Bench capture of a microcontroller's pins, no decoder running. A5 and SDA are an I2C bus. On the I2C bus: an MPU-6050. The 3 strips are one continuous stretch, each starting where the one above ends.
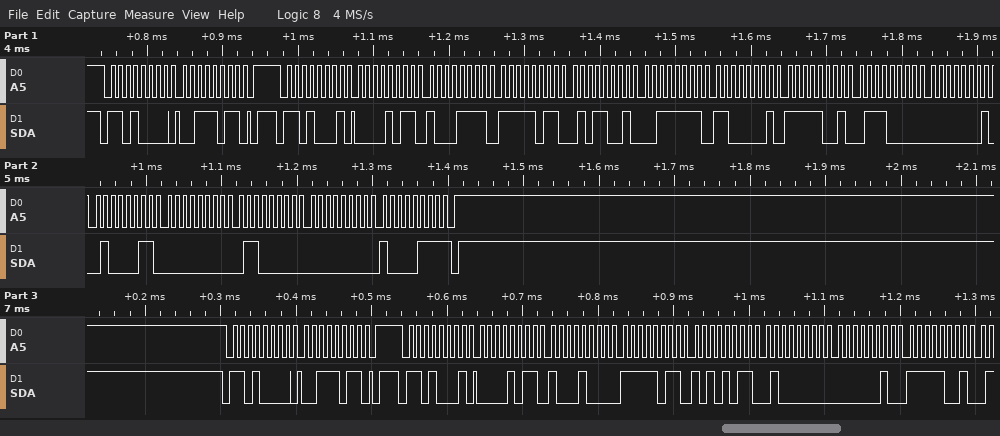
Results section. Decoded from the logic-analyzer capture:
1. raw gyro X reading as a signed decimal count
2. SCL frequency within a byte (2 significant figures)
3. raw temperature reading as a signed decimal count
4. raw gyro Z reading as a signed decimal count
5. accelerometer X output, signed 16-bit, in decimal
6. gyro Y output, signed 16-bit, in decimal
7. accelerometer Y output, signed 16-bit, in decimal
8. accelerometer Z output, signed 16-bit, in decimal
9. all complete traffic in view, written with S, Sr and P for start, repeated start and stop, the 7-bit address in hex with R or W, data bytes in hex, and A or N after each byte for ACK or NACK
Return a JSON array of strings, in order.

["323", "100 kHz", "-1680", "135", "2959", "96", "-1191", "16321", "S 68W A 3B A P S 68R A 0B A 8F A FB A 59 A 3F A C1 A F9 A 70 A 01 A 43 A 00 A 60 A 00 A 87 N P S 68W A 3B A P S 68R A 0B A 88 A FB A AB A 40 A 02 A F9 A"]
